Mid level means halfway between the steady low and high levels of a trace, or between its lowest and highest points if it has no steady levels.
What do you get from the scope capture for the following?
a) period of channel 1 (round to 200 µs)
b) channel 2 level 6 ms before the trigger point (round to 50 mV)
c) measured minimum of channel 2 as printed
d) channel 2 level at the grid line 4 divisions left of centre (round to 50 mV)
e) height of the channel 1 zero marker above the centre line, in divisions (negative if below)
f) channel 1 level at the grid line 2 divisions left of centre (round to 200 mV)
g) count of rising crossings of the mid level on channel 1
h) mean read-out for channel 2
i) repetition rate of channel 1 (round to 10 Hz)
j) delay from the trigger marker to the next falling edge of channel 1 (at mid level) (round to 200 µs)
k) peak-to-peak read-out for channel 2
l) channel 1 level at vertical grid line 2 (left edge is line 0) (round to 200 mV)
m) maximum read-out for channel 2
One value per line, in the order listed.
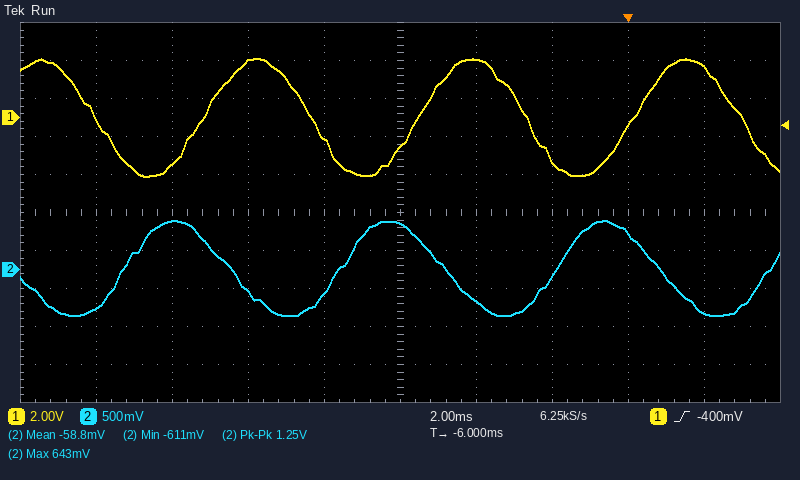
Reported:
5.6 ms
600 mV
-611 mV
-500 mV
+2.5 div
3.0 V
3
-58.8 mV
180 Hz
3.0 ms
1.25 V
-2.4 V
643 mV
